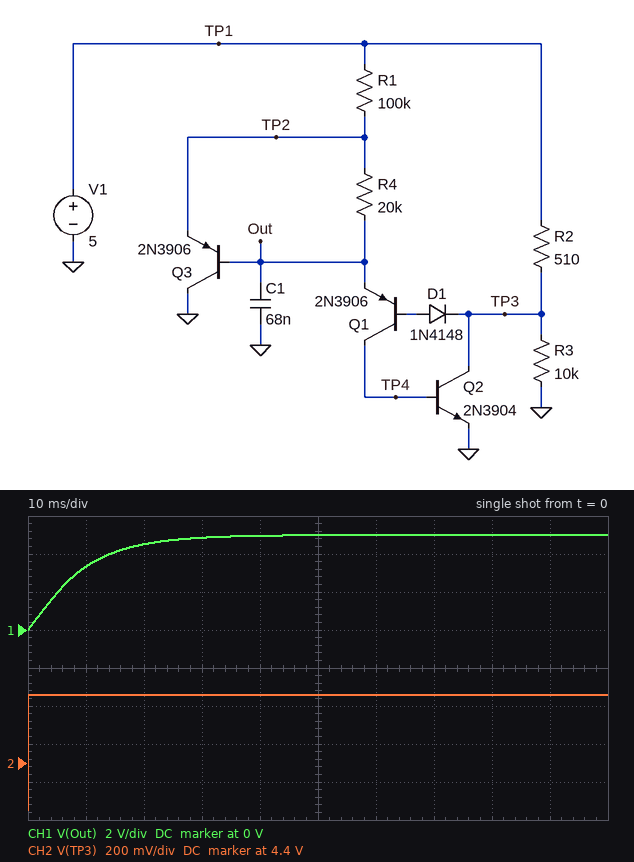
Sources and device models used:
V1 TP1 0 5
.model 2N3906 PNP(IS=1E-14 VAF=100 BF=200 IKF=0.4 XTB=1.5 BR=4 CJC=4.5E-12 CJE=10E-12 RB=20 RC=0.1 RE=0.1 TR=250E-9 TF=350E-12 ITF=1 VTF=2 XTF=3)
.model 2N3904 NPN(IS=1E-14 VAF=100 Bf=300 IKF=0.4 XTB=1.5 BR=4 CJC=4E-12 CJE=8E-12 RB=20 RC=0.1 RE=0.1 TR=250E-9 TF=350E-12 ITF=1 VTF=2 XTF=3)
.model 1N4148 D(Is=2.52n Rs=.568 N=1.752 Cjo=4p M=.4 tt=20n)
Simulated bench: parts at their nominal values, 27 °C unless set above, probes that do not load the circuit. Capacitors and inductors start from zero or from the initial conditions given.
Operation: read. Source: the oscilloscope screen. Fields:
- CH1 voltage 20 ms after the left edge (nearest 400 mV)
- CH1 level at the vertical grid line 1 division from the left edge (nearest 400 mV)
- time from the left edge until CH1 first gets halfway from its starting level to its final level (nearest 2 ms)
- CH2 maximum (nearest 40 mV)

4.4 V
3.2 V
6 ms
4.76 V
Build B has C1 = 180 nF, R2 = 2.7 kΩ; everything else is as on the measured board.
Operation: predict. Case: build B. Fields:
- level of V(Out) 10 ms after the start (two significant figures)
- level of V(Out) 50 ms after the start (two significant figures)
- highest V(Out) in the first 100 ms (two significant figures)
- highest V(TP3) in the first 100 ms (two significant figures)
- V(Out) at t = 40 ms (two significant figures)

1.5 V
830 mV
4.3 V
3.9 V
4.1 V
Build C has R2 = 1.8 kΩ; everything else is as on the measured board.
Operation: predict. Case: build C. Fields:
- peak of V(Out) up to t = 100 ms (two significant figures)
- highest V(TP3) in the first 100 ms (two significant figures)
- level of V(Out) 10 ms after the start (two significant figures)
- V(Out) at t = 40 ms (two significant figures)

4.6 V
4.2 V
3.3 V
4.5 V
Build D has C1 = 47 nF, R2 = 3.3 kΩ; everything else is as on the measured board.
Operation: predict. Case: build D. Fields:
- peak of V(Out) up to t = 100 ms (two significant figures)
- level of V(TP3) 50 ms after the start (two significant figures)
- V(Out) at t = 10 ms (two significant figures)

4.2 V
3.8 V
4.0 V
